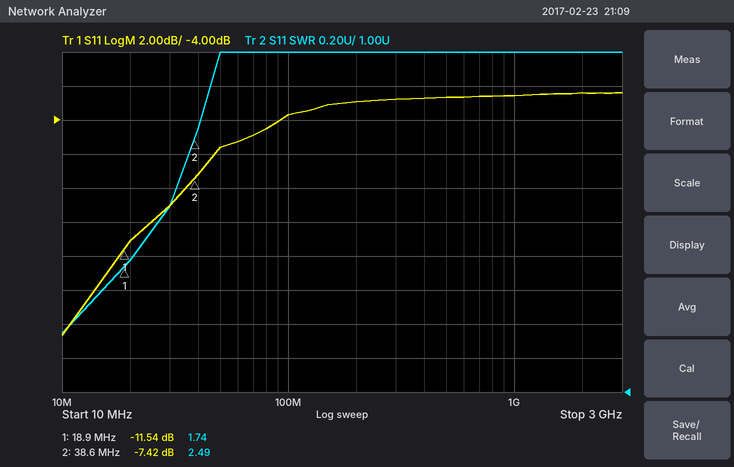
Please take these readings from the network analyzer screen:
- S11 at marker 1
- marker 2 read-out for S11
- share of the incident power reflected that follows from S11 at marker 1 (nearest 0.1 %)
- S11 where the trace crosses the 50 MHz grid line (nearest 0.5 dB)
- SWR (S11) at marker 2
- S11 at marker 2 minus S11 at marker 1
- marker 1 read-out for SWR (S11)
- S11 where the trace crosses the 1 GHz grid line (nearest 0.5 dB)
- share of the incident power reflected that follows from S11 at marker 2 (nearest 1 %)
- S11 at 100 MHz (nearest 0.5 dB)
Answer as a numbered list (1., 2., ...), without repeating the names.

1. -11.54 dB
2. -7.42 dB
3. 7.0 %
4. -5.5 dB
5. 2.49
6. 4.12 dB
7. 1.74
8. -2.5 dB
9. 18 %
10. -3.5 dB
